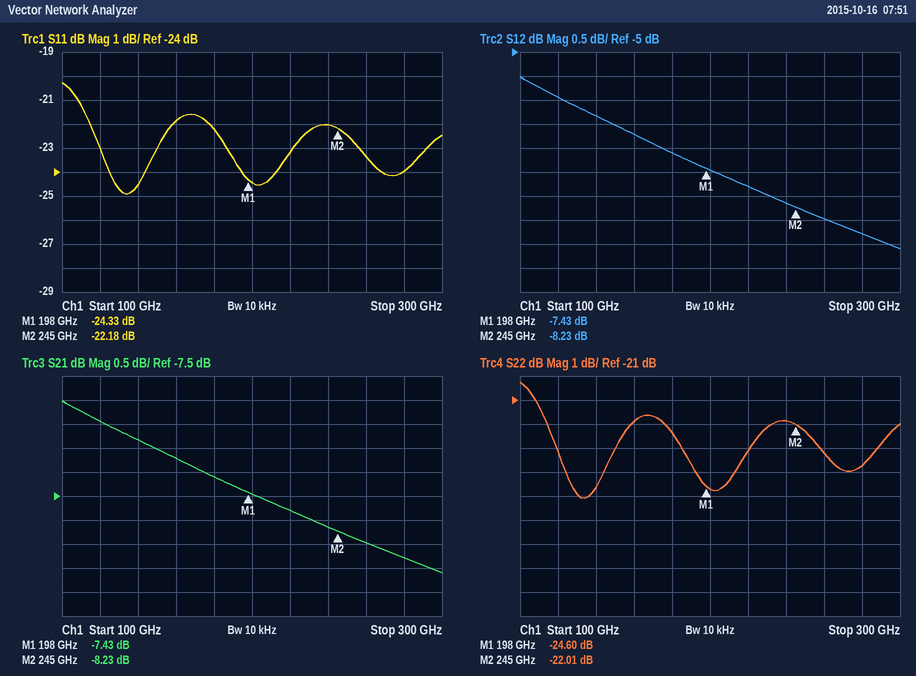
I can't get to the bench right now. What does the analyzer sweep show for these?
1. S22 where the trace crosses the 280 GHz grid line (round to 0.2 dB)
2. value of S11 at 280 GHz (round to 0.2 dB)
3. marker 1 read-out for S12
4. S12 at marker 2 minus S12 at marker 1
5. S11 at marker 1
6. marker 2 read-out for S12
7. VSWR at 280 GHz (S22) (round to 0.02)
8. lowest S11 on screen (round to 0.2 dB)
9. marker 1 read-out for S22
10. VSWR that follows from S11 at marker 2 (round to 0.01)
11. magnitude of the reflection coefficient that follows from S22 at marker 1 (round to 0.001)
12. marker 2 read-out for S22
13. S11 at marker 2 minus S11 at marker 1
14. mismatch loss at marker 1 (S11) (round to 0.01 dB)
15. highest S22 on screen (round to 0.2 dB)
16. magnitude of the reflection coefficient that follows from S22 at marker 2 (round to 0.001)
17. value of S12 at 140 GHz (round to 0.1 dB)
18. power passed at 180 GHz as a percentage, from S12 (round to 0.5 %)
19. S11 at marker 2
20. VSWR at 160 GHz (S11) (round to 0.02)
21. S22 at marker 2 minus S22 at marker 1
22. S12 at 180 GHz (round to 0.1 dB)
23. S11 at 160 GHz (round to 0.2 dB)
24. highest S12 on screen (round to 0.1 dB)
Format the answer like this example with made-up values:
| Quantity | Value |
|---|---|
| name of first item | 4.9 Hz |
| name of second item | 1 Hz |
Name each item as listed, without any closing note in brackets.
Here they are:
| Quantity | Value |
|---|---|
| S22 where the trace crosses the 280 GHz grid line | -23.8 dB |
| value of S11 at 280 GHz | -24.0 dB |
| marker 1 read-out for S12 | -7.43 dB |
| S12 at marker 2 minus S12 at marker 1 | -0.80 dB |
| S11 at marker 1 | -24.33 dB |
| marker 2 read-out for S12 | -8.23 dB |
| VSWR at 280 GHz (S22) | 1.14 |
| lowest S11 on screen | -25.0 dB |
| marker 1 read-out for S22 | -24.60 dB |
| VSWR that follows from S11 at marker 2 | 1.17 |
| magnitude of the reflection coefficient that follows from S22 at marker 1 | 0.059 |
| marker 2 read-out for S22 | -22.01 dB |
| S11 at marker 2 minus S11 at marker 1 | 2.15 dB |
| mismatch loss at marker 1 (S11) | 0.02 dB |
| highest S22 on screen | -20.2 dB |
| magnitude of the reflection coefficient that follows from S22 at marker 2 | 0.079 |
| value of S12 at 140 GHz | -6.3 dB |
| power passed at 180 GHz as a percentage, from S12 | 19.5 % |
| S11 at marker 2 | -22.18 dB |
| VSWR at 160 GHz (S11) | 1.18 |
| S22 at marker 2 minus S22 at marker 1 | 2.59 dB |
| S12 at 180 GHz | -7.1 dB |
| S11 at 160 GHz | -21.8 dB |
| highest S12 on screen | -5.5 dB |
